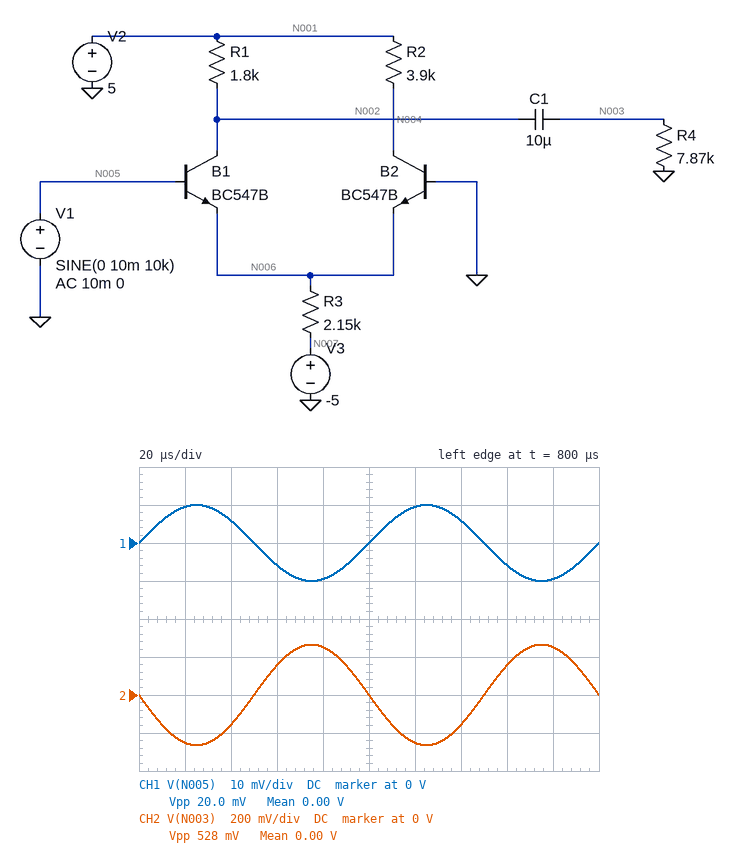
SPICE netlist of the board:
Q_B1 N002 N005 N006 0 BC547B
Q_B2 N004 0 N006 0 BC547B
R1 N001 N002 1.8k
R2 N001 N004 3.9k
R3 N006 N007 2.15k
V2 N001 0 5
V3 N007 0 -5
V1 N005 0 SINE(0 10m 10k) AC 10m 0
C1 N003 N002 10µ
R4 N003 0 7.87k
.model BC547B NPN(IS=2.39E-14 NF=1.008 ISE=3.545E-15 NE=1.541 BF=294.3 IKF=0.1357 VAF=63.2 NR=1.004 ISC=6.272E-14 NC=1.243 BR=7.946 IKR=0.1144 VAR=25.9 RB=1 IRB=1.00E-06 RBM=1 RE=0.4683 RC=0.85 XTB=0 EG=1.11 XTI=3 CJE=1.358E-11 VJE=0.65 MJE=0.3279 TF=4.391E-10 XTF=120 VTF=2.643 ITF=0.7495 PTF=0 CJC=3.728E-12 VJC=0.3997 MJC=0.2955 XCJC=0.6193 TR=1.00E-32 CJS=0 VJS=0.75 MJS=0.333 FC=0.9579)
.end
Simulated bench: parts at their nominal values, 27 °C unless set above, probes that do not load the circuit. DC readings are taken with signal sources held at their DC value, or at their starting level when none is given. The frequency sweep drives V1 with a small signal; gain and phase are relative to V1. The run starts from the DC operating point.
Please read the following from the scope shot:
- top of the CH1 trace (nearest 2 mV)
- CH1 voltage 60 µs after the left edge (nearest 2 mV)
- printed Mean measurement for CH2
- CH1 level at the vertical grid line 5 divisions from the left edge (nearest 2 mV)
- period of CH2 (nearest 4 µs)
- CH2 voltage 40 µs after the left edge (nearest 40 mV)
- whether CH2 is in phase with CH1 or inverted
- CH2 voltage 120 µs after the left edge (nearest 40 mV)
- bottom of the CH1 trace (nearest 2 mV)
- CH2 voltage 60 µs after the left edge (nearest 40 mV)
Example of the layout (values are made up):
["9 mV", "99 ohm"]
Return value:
["10 mV", "-6 mV", "0.00 V", "0 V", "100 µs", "-160 mV", "inverted", "-240 mV", "-10 mV", "160 mV"]
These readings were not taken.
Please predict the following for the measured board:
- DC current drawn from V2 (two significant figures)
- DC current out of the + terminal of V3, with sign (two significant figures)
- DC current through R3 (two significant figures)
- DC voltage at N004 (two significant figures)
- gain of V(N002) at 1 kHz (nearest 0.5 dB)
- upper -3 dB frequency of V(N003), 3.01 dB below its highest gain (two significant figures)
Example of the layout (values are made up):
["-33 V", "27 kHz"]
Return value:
["2.0 mA", "-2.0 mA", "2.0 mA", "1.1 V", "28.5 dB", "58 MHz"]
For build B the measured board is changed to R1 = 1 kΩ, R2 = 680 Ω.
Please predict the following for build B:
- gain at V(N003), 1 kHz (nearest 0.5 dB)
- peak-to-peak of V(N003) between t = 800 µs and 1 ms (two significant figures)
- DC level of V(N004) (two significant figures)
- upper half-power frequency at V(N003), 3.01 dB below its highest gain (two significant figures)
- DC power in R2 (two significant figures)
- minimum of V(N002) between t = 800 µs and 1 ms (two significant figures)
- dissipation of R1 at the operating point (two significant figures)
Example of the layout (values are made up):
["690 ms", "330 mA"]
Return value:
["24.5 dB", "330 mV", "4.3 V", "96 MHz", "700 µW", "3.8 V", "1.0 mW"]
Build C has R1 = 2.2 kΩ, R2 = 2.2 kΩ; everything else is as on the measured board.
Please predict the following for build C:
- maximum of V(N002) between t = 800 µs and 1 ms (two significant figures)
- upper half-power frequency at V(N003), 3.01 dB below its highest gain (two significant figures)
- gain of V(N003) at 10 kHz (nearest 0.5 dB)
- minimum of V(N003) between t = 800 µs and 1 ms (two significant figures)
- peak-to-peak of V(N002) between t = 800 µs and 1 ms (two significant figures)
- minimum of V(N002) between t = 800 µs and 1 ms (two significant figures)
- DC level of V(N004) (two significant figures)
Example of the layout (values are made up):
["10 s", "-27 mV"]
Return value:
["3.1 V", "46 MHz", "30.0 dB", "-310 mV", "630 mV", "2.5 V", "2.8 V"]
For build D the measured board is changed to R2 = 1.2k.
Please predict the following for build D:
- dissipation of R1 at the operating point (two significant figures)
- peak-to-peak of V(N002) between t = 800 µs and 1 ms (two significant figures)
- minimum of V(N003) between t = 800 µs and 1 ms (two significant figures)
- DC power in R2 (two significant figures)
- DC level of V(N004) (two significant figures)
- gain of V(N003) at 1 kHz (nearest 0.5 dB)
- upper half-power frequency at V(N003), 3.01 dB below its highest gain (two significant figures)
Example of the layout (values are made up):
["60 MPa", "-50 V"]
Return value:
["1.8 mW", "540 mV", "-270 mV", "1.2 mW", "3.8 V", "28.5 dB", "55 MHz"]
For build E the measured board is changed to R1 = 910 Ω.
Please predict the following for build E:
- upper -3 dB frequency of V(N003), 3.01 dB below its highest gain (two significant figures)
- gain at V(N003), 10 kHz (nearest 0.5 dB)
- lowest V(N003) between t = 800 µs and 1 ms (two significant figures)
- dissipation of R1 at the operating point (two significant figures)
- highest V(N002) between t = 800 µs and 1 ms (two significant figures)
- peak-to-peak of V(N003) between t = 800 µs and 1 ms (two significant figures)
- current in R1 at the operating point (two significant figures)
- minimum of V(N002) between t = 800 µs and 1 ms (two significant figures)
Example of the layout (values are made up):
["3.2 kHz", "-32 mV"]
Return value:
["110 MHz", "23.5 dB", "-150 mV", "970 µW", "4.2 V", "300 mV", "1.0 mA", "3.9 V"]
